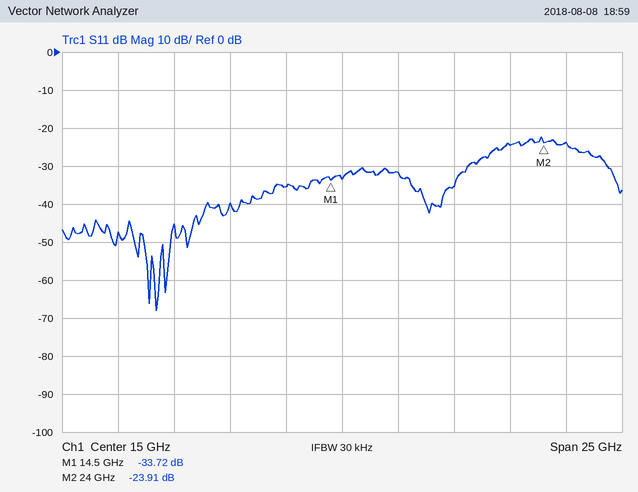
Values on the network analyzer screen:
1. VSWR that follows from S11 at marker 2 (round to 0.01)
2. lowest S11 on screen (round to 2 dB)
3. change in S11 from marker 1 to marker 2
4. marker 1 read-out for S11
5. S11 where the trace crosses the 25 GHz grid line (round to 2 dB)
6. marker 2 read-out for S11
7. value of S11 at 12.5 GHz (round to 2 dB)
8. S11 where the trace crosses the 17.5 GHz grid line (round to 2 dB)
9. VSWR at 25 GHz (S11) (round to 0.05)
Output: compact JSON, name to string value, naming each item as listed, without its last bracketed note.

{"VSWR that follows from S11 at marker 2": "1.14", "lowest S11 on screen": "-68 dB", "change in S11 from marker 1 to marker 2": "9.81 dB", "marker 1 read-out for S11": "-33.72 dB", "S11 where the trace crosses the 25 GHz grid line": "-24 dB", "marker 2 read-out for S11": "-23.91 dB", "value of S11 at 12.5 GHz": "-36 dB", "S11 where the trace crosses the 17.5 GHz grid line": "-32 dB", "VSWR at 25 GHz (S11)": "1.15"}
